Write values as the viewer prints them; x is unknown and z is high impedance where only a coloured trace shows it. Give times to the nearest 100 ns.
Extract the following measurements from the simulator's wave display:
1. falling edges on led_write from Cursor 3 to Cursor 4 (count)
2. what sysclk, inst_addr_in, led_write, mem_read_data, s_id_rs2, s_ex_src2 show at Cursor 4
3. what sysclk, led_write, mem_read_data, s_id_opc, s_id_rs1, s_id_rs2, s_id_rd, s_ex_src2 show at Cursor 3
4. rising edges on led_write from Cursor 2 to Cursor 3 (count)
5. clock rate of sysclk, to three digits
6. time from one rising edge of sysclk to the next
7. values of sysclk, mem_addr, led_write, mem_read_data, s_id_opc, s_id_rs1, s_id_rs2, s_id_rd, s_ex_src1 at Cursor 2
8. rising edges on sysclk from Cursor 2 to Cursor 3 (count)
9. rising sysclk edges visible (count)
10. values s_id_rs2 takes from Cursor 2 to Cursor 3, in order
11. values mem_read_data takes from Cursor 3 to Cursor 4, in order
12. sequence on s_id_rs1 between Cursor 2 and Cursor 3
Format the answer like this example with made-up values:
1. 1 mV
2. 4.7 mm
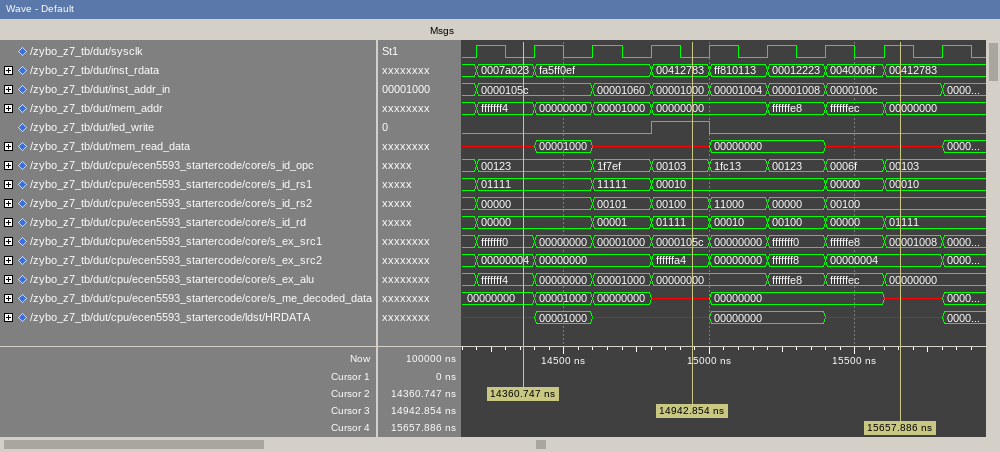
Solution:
1. 1
2. sysclk=1, inst_addr_in=0000100c, led_write=0, mem_read_data=x, s_id_rs2=00100, s_ex_src2=00000004
3. sysclk=0, led_write=1, mem_read_data=x, s_id_opc=00103, s_id_rs1=00010, s_id_rs2=00100, s_id_rd=01111, s_ex_src2=ffffffa4
4. 1
5. 5.00 MHz
6. 200 ns
7. sysclk=0, mem_addr=fffffff4, led_write=0, mem_read_data=x, s_id_opc=00123, s_id_rs1=01111, s_id_rs2=00000, s_id_rd=00000, s_ex_src1=fffffff0
8. 3
9. 9
10. 00000, 00101, 00100
11. x, 00000000, x
12. 01111, 11111, 00010
